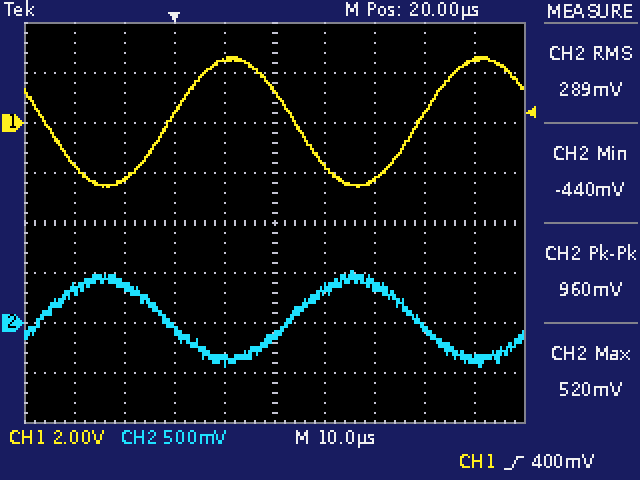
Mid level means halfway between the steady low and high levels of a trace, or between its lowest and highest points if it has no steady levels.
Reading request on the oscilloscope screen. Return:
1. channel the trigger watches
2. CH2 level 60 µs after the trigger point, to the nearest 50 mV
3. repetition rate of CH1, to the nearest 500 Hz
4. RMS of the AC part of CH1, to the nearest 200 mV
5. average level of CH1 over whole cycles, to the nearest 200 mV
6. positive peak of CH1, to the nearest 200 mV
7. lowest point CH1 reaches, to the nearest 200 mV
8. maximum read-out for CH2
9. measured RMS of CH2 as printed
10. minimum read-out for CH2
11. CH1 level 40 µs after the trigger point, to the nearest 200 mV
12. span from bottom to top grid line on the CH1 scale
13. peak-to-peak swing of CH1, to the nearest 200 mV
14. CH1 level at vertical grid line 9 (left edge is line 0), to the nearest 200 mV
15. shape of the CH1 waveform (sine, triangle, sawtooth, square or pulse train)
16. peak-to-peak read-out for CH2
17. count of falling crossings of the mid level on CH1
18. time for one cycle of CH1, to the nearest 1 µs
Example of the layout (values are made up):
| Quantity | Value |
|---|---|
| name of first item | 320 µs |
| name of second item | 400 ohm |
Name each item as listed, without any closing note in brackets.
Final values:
| Quantity | Value |
|---|---|
| channel the trigger watches | CH1 |
| CH2 level 60 µs after the trigger point, to the nearest 50 mV | -350 mV |
| repetition rate of CH1, to the nearest 500 Hz | 20.0 kHz |
| RMS of the AC part of CH1, to the nearest 200 mV | 1.8 V |
| average level of CH1 over whole cycles, to the nearest 200 mV | 0.0 V |
| positive peak of CH1, to the nearest 200 mV | 2.6 V |
| lowest point CH1 reaches, to the nearest 200 mV | -2.6 V |
| maximum read-out for CH2 | 520 mV |
| measured RMS of CH2 as printed | 289 mV |
| minimum read-out for CH2 | -440 mV |
| CH1 level 40 µs after the trigger point, to the nearest 200 mV | -2.2 V |
| span from bottom to top grid line on the CH1 scale | 16 V |
| peak-to-peak swing of CH1, to the nearest 200 mV | 5.2 V |
| CH1 level at vertical grid line 9 (left edge is line 0), to the nearest 200 mV | 2.6 V |
| shape of the CH1 waveform | sine |
| peak-to-peak read-out for CH2 | 960 mV |
| count of falling crossings of the mid level on CH1 | 2 |
| time for one cycle of CH1, to the nearest 1 µs | 50 µs |
